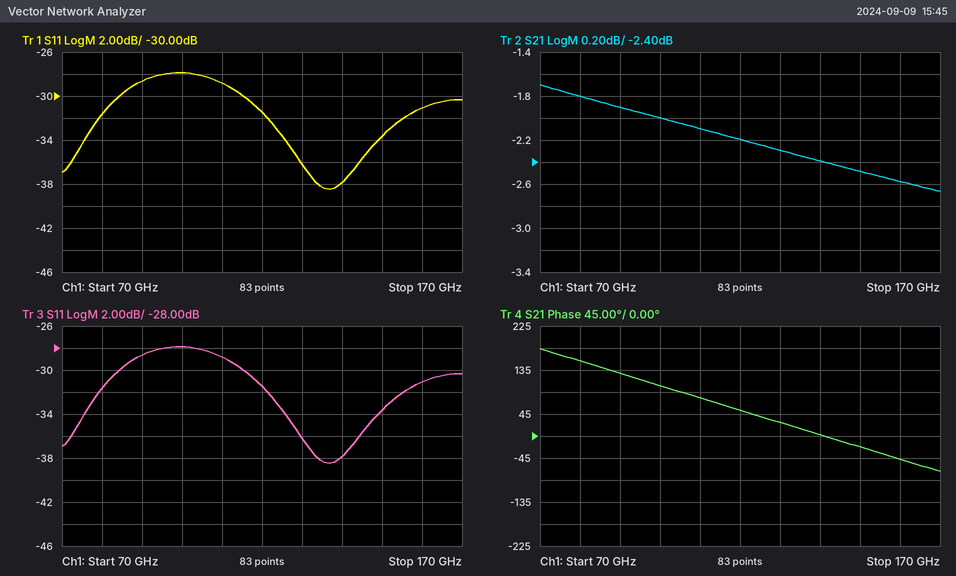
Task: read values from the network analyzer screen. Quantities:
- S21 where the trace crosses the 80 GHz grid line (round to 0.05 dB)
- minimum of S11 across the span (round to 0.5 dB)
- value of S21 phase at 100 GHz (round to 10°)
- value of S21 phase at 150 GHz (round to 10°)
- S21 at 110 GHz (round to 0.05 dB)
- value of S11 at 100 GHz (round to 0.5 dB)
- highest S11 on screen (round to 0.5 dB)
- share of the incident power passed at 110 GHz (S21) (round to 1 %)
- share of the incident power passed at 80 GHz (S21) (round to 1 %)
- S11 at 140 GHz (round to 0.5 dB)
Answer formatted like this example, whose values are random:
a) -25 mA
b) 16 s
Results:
a) -1.80 dB
b) -38.5 dB
c) 100°
d) -20°
e) -2.10 dB
f) -28.0 dB
g) -28.0 dB
h) 62 %
i) 66 %
j) -38.0 dB
